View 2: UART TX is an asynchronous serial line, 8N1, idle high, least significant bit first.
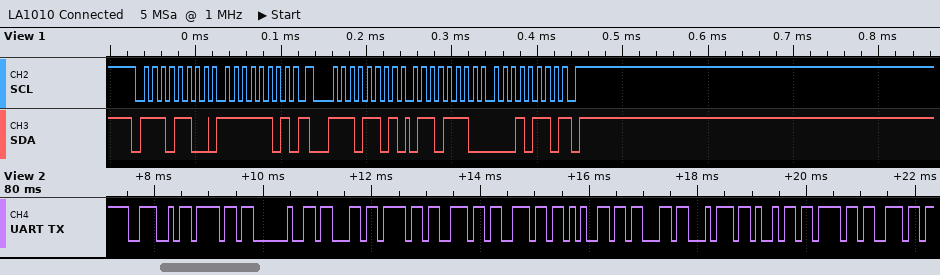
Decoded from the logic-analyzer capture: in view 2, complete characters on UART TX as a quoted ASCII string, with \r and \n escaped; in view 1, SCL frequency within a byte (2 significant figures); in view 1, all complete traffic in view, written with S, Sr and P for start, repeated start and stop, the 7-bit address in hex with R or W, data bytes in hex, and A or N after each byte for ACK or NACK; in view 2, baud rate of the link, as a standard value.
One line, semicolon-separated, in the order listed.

"No connection"; 100 kHz; S 76W A FD A Sr 76R A 6E A 16 N P; 9600 baud
